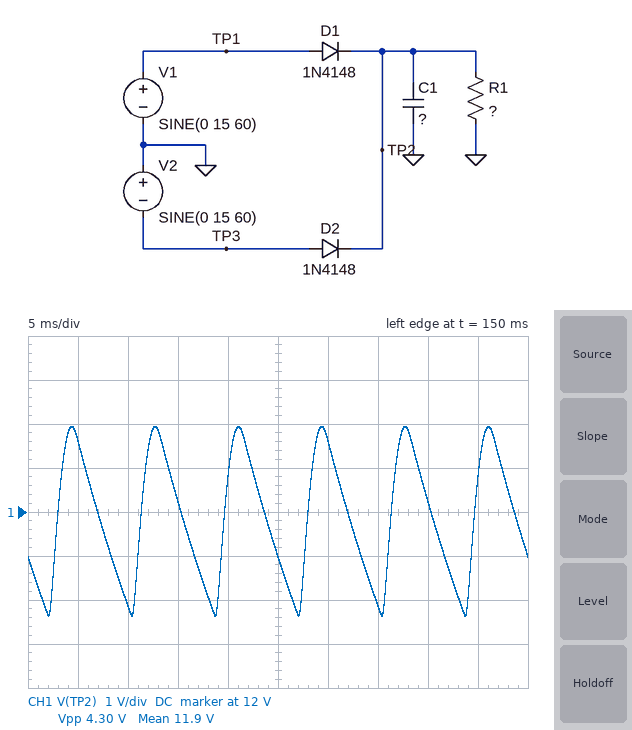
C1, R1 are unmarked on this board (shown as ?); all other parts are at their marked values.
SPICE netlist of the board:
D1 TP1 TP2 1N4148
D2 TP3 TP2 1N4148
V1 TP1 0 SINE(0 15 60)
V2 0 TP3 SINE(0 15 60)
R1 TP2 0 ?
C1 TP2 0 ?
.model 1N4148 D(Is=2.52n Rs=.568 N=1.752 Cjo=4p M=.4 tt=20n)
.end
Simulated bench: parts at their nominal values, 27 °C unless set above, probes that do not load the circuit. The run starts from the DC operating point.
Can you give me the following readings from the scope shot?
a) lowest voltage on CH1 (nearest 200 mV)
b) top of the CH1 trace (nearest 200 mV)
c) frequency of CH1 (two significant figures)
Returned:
9.6 V
14.0 V
120 Hz
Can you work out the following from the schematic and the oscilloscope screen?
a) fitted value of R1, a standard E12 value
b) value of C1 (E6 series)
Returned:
47 Ω
330 µF
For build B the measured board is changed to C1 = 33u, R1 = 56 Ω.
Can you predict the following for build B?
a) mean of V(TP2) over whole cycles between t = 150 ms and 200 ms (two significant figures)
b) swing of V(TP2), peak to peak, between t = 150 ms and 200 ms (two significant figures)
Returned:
9.1 V
12 V
